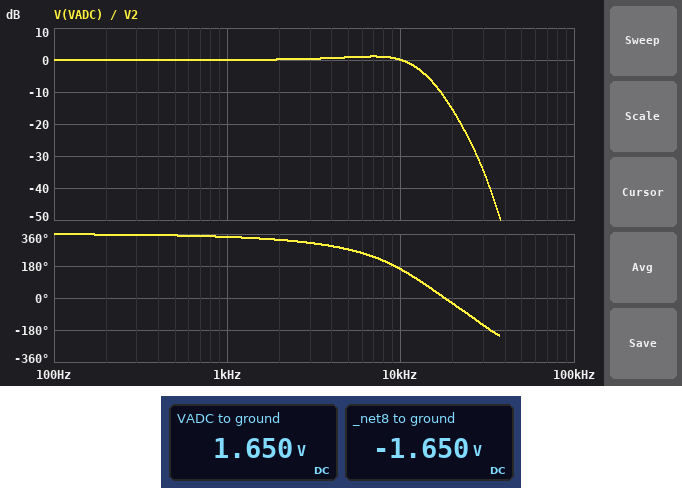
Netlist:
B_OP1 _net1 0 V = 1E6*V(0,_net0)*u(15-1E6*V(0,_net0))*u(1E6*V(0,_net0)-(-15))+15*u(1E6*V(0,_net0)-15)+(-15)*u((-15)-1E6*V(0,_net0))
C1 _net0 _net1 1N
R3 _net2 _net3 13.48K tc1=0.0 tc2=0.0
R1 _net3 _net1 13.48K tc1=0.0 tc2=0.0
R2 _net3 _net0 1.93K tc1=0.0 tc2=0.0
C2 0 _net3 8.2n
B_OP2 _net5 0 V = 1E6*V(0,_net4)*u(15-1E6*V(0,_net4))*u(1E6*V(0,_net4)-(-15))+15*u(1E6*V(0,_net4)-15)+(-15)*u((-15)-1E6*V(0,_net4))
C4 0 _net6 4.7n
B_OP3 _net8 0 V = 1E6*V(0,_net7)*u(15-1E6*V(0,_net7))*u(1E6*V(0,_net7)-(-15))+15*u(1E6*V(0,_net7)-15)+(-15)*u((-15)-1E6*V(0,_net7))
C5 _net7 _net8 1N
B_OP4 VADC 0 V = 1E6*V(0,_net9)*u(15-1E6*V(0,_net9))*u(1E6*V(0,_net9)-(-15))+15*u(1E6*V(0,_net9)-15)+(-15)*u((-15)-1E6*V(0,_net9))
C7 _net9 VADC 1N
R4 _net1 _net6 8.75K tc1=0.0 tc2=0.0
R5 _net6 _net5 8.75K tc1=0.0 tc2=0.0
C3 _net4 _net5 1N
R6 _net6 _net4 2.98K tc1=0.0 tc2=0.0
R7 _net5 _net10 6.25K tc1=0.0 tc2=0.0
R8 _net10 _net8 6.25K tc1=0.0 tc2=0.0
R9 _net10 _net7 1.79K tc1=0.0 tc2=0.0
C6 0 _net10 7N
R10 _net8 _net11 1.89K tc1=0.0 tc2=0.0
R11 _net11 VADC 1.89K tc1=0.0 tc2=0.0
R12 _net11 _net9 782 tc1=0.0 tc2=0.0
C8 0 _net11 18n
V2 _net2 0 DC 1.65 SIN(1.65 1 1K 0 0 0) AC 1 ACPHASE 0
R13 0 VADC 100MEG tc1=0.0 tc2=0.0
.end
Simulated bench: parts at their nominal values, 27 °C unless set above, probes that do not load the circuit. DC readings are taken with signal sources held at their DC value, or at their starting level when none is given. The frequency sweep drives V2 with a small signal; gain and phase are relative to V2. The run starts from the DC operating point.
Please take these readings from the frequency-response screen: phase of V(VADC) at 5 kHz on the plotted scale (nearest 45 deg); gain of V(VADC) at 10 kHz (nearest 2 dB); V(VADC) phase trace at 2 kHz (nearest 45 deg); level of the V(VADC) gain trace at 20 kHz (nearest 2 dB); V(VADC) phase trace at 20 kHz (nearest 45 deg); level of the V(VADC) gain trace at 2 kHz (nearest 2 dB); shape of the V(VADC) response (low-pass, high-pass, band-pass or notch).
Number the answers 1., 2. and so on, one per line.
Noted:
1. 270 deg
2. 0 dB
3. 315 deg
4. -16 dB
5. -45 deg
6. 0 dB
7. low-pass
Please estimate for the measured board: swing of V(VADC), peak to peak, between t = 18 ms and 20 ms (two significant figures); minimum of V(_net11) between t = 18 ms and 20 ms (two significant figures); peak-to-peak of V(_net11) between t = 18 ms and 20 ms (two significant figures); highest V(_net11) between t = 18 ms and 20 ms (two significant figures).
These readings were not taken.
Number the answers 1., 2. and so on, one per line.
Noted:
1. 2.0 V
2. -4.9 mV
3. 9.9 mV
4. 4.9 mV
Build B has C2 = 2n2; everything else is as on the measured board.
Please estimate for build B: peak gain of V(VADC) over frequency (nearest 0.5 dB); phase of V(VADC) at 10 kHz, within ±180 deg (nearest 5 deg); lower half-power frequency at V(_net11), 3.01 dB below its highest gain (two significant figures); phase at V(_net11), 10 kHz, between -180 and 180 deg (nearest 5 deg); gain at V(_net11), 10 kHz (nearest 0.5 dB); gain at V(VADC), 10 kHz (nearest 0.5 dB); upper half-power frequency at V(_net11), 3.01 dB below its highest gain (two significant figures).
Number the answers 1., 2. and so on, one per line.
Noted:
1. 0 dB
2. -170 deg
3. 6.5 kHz
4. 100 deg
5. -28.0 dB
6. -1.5 dB
7. 18 kHz
